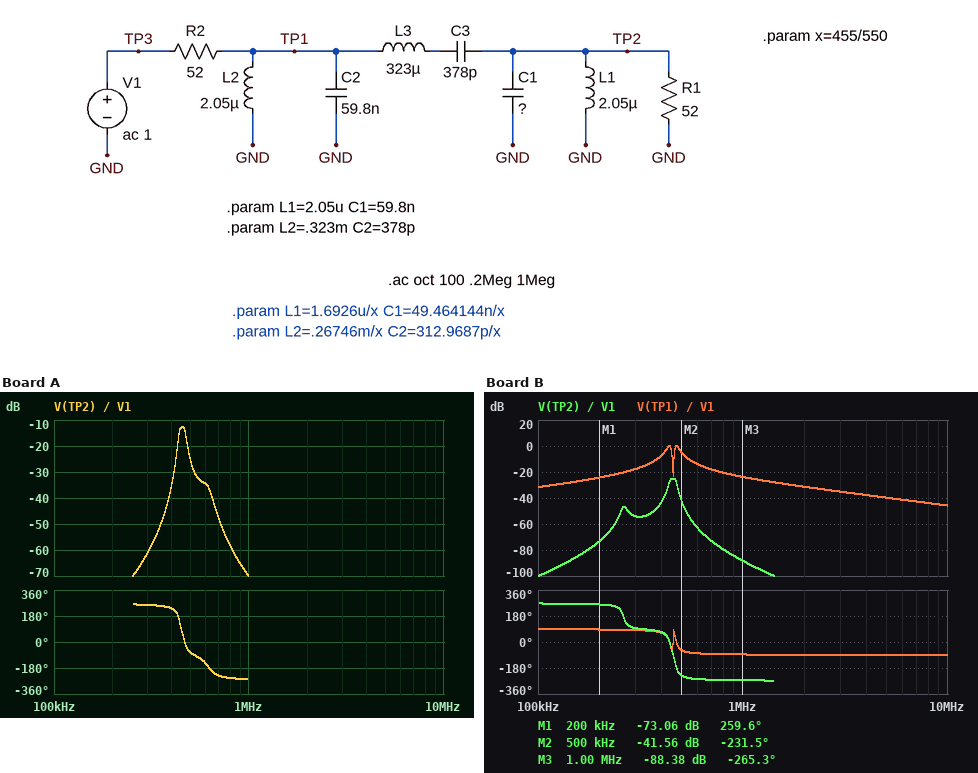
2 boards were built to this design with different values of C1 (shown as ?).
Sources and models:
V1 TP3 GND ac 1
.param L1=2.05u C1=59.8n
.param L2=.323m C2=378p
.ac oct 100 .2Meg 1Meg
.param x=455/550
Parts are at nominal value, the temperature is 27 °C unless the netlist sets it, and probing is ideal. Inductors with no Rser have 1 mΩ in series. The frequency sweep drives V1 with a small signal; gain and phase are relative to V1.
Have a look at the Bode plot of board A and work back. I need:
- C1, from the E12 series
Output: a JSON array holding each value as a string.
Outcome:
["33 nF"]
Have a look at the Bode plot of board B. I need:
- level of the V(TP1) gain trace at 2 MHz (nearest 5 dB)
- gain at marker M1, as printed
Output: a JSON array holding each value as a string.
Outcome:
["-30 dB", "-73.06 dB"]
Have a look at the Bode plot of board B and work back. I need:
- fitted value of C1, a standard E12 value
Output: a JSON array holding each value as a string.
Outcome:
["180 nF"]
